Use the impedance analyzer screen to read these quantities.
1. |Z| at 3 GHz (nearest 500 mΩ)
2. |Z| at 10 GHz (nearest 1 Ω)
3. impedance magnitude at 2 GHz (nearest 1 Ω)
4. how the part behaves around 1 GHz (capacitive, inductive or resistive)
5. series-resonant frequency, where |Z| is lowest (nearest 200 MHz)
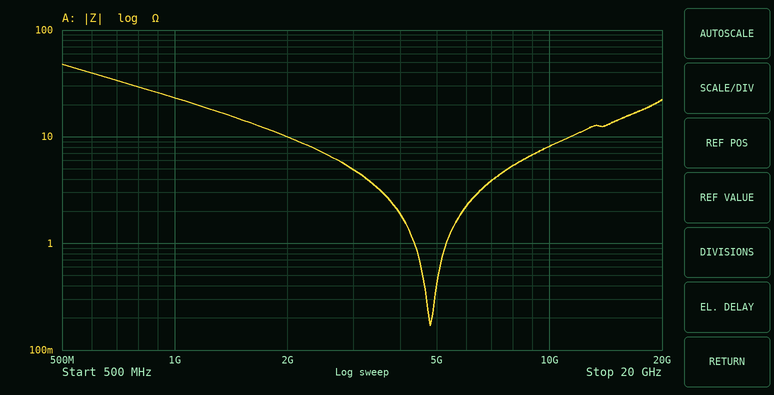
5.0 Ω
8 Ω
10 Ω
capacitive
4.8 GHz
